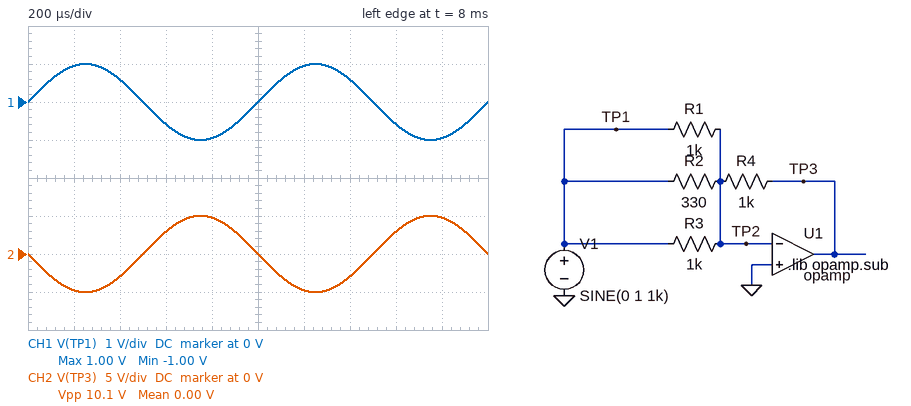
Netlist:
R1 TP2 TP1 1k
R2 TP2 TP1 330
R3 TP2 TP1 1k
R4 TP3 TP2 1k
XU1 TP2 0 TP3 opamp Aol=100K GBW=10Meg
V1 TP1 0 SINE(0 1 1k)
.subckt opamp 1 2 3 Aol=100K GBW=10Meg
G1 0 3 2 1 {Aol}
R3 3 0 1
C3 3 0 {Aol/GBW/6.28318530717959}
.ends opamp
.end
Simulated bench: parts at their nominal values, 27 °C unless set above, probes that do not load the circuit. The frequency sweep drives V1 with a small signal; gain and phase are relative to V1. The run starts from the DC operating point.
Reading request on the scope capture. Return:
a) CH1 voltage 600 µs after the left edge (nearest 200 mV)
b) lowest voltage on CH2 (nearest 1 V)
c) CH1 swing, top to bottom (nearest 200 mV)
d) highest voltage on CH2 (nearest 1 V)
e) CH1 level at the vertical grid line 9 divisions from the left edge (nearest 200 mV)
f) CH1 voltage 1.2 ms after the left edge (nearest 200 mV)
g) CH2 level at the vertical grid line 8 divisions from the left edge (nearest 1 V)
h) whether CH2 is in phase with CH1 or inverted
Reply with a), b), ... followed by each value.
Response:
a) -600 mV
b) -5 V
c) 2.0 V
d) 5 V
e) -1.0 V
f) 1.0 V
g) 3 V
h) inverted
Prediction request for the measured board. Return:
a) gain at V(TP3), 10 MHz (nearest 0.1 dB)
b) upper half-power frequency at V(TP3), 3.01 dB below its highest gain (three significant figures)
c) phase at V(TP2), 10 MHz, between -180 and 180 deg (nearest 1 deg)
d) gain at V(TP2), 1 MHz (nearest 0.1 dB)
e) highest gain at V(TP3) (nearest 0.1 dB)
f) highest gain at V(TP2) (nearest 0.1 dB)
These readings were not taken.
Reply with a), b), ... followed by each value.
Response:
a) -1.7 dB
b) 1.66 MHz
c) 9 deg
d) -7.3 dB
e) 14.0 dB
f) -1.6 dB
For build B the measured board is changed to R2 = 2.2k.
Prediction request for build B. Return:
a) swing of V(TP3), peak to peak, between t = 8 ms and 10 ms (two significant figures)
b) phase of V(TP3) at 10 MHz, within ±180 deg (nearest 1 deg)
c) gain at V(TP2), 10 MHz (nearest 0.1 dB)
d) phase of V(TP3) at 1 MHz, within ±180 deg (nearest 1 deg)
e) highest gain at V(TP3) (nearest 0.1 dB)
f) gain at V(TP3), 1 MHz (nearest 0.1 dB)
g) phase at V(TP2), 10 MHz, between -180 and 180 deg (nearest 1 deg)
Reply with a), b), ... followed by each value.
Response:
a) 4.9 V
b) 106 deg
c) -3.3 dB
d) 161 deg
e) 7.8 dB
f) 7.3 dB
g) 16 deg
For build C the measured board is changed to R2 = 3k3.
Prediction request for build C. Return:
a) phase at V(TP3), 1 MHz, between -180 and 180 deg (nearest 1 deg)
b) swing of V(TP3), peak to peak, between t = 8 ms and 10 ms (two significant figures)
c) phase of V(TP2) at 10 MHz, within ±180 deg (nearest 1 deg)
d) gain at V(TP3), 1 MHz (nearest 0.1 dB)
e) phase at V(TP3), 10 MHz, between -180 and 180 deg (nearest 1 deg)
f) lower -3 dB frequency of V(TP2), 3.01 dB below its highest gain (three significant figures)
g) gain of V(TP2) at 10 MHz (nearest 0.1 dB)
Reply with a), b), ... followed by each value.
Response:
a) 162 deg
b) 4.6 V
c) 17 deg
d) 6.8 dB
e) 107 deg
f) 3.03 MHz
g) -3.5 dB
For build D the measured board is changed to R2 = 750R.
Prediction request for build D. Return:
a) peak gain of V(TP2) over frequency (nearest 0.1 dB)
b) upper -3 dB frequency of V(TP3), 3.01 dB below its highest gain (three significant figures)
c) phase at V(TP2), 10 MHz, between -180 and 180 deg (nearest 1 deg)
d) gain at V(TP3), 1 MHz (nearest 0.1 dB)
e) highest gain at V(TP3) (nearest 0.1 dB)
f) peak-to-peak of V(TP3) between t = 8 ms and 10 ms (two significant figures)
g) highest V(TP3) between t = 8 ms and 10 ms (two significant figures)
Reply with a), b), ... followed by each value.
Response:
a) -2.3 dB
b) 2.31 MHz
c) 13 deg
d) 9.7 dB
e) 10.5 dB
f) 6.7 V
g) 3.3 V
